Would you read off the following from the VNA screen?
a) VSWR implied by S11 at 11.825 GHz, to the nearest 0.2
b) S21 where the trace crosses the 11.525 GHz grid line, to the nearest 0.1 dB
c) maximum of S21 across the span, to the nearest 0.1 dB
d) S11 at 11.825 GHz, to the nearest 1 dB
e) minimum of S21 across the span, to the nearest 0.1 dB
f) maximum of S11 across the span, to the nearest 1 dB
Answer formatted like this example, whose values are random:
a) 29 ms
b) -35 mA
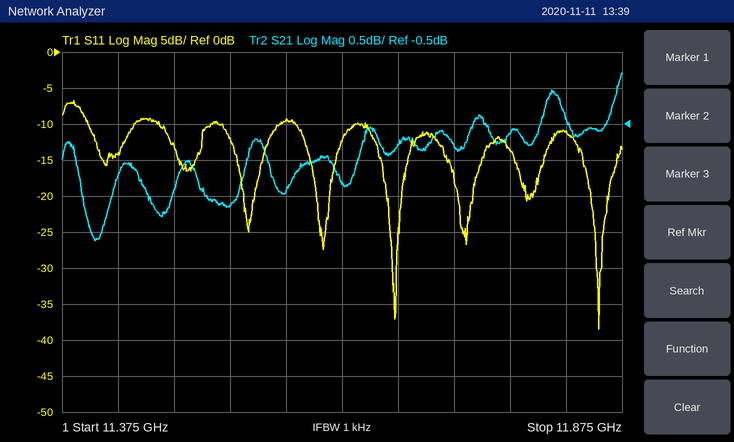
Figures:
a) 1.8
b) -1.6 dB
c) 0.2 dB
d) -11 dB
e) -2.1 dB
f) -7 dB
